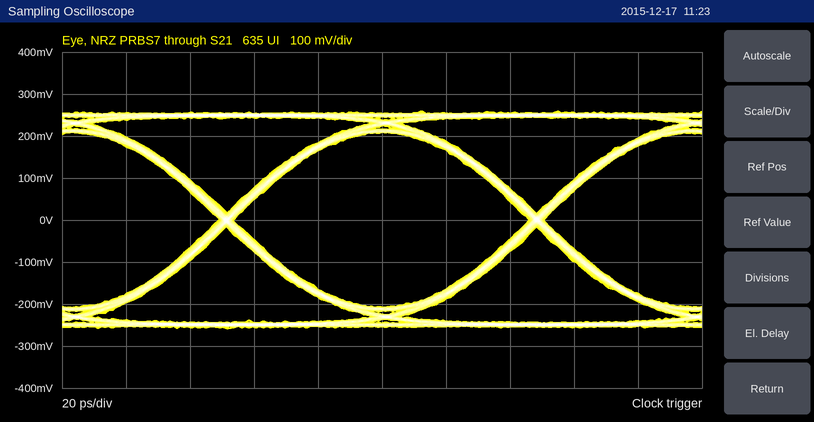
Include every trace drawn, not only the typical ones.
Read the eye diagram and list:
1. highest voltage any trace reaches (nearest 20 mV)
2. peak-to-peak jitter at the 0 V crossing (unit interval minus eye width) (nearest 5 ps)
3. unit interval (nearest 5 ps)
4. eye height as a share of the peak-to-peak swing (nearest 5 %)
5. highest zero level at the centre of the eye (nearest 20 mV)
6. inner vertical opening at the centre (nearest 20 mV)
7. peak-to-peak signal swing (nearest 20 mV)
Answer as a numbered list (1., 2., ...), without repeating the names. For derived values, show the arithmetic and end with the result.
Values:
1. 260 mV
2. 5 ps
3. 95 ps
4. 420 mV / 520 mV ≈ 80.8 %, so 80 % to the nearest 5 %
5. -200 mV
6. 420 mV
7. 520 mV
